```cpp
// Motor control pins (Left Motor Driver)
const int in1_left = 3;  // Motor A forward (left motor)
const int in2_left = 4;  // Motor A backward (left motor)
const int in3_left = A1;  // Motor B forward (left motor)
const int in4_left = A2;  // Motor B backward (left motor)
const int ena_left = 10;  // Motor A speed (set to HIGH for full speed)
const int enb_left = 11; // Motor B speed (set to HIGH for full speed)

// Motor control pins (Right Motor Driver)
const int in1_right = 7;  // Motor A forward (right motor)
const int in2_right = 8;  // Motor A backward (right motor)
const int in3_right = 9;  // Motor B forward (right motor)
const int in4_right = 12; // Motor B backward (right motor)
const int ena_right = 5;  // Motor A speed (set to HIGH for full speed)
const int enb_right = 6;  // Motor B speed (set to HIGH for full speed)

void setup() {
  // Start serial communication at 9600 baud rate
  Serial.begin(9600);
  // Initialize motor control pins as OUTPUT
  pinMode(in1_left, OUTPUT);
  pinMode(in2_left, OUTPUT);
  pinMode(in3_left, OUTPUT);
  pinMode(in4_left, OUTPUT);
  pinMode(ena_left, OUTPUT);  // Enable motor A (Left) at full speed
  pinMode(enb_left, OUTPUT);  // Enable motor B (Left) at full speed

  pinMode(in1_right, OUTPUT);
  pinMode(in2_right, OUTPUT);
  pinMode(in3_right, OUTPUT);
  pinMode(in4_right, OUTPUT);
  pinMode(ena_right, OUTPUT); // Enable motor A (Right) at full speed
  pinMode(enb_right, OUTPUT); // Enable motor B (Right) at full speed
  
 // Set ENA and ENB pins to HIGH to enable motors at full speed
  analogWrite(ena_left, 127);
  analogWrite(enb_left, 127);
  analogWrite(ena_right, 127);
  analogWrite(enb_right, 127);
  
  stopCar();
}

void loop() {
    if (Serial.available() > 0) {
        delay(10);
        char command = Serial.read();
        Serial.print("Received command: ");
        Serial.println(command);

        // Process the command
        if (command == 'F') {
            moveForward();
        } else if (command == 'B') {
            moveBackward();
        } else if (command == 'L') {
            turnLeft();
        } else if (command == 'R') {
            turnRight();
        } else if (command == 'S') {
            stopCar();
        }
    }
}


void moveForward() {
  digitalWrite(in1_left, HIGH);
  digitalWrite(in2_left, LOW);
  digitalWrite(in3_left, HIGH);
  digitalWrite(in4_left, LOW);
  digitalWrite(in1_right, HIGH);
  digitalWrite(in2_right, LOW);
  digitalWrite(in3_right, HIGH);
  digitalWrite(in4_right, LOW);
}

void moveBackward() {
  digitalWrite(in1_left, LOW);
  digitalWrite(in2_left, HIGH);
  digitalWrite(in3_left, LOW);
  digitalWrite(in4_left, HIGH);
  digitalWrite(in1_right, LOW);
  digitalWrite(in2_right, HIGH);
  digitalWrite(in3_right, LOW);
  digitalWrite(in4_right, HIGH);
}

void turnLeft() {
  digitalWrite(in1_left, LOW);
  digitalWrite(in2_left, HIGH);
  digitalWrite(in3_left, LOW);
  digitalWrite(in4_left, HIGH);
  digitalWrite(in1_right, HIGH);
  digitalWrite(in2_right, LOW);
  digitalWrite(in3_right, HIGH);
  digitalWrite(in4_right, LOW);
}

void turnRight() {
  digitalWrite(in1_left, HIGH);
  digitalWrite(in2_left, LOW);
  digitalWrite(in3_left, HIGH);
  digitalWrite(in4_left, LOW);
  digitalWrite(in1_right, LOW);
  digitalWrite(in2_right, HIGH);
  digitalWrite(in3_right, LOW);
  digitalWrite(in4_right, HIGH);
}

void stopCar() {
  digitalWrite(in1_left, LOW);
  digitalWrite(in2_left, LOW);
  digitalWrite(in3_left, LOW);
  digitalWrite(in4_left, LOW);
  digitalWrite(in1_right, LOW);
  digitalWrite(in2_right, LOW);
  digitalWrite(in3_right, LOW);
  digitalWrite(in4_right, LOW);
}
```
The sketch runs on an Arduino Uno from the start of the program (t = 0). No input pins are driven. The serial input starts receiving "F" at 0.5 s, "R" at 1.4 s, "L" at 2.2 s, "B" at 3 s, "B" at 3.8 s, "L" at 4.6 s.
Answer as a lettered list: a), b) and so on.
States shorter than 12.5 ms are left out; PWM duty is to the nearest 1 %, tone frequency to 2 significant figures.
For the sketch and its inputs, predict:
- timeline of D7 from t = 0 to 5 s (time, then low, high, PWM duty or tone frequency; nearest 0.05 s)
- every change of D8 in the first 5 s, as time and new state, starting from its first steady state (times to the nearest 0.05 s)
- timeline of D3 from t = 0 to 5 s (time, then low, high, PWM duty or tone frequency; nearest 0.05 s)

a) 0 s low; 0.5 s high; 1.4 s low; 2.2 s high; 3 s low; 4.6 s high
b) 0 s low; 1.4 s high; 2.2 s low; 3 s high; 4.6 s low
c) 0 s low; 0.5 s high; 2.2 s low
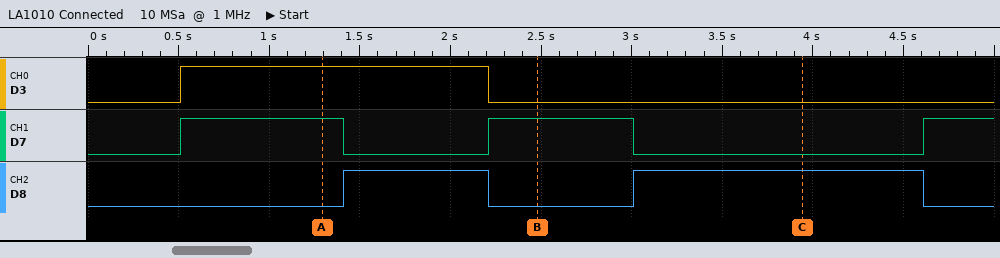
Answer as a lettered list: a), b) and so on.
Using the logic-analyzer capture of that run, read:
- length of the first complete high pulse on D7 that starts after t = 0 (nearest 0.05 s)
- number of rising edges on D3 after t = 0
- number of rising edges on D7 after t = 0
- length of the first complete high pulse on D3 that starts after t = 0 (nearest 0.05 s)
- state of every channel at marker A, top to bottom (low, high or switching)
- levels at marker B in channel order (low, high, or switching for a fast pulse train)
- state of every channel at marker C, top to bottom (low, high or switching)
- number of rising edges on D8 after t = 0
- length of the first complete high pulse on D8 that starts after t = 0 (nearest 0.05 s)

a) 0.90 s
b) 1
c) 3
d) 1.70 s
e) D3 high, D7 high, D8 low
f) D3 low, D7 high, D8 low
g) D3 low, D7 low, D8 high
h) 2
i) 0.80 s
